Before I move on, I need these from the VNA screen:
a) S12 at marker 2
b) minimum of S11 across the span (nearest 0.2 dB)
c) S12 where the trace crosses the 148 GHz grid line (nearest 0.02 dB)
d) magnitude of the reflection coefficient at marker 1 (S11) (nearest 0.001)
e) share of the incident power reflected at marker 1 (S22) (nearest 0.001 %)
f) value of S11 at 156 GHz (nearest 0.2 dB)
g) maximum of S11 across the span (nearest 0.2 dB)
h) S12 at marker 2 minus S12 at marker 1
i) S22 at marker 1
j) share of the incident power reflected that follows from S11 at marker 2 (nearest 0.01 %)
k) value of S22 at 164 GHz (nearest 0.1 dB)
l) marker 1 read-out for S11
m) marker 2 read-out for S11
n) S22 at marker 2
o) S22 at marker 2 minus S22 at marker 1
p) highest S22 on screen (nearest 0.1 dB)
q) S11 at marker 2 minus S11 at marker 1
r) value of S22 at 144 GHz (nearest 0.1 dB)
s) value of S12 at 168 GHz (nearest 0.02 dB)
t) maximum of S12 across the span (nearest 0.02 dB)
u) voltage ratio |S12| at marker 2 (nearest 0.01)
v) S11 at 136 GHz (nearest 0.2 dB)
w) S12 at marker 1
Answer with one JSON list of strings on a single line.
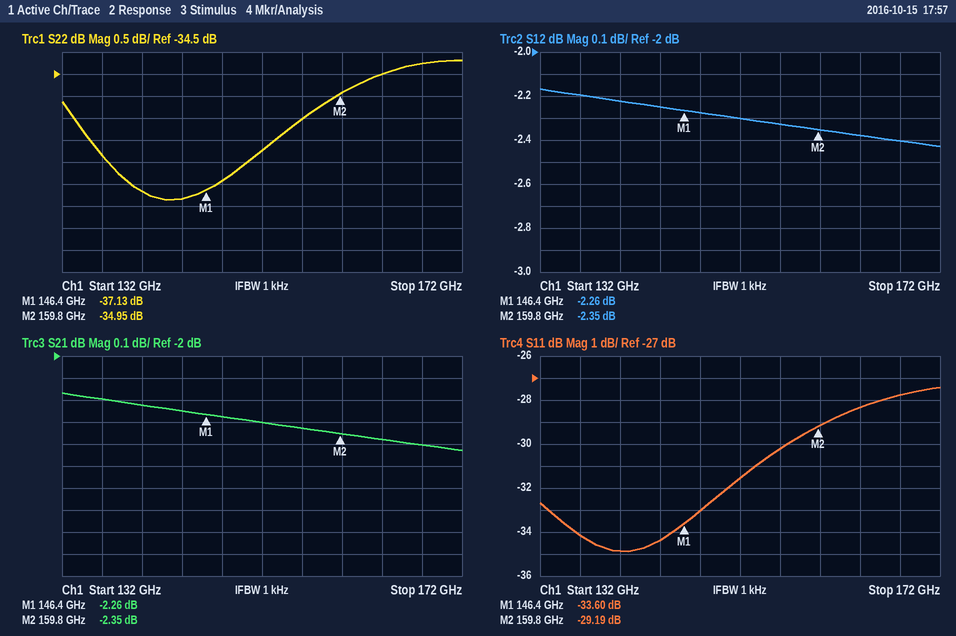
["-2.35 dB", "-34.8 dB", "-2.28 dB", "0.021", "0.019 %", "-30.2 dB", "-27.4 dB", "-0.09 dB", "-37.13 dB", "0.12 %", "-34.5 dB", "-33.60 dB", "-29.19 dB", "-34.95 dB", "2.18 dB", "-34.2 dB", "4.41 dB", "-37.3 dB", "-2.40 dB", "-2.16 dB", "0.76", "-34.2 dB", "-2.26 dB"]
